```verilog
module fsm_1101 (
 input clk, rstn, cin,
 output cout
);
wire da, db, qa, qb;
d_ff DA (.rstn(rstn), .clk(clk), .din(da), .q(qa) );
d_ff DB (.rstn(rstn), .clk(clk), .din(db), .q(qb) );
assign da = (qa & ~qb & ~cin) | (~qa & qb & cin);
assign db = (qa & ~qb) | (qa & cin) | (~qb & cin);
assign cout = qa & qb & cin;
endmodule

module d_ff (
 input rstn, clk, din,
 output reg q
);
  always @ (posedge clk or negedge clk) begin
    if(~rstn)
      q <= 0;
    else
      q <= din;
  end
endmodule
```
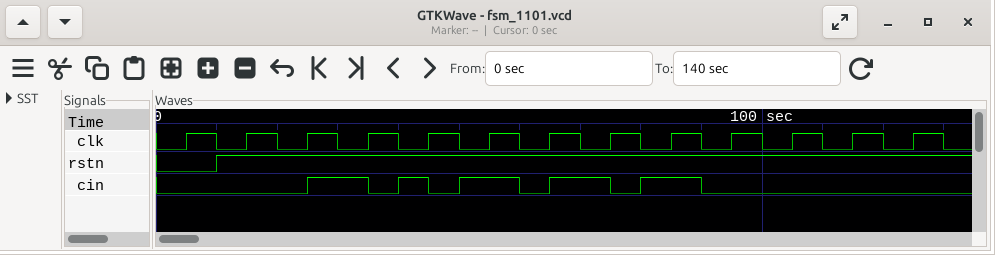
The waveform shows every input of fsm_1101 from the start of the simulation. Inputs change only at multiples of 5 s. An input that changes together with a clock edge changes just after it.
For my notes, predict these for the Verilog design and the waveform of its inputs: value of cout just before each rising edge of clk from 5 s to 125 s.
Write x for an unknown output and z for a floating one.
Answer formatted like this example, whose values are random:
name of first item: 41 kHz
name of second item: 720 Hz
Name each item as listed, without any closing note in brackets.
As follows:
value of cout just before each rising edge of clk from 5 s to 125 s: 0 0 0 0 1 0 0 0 1 0 0 0 0
